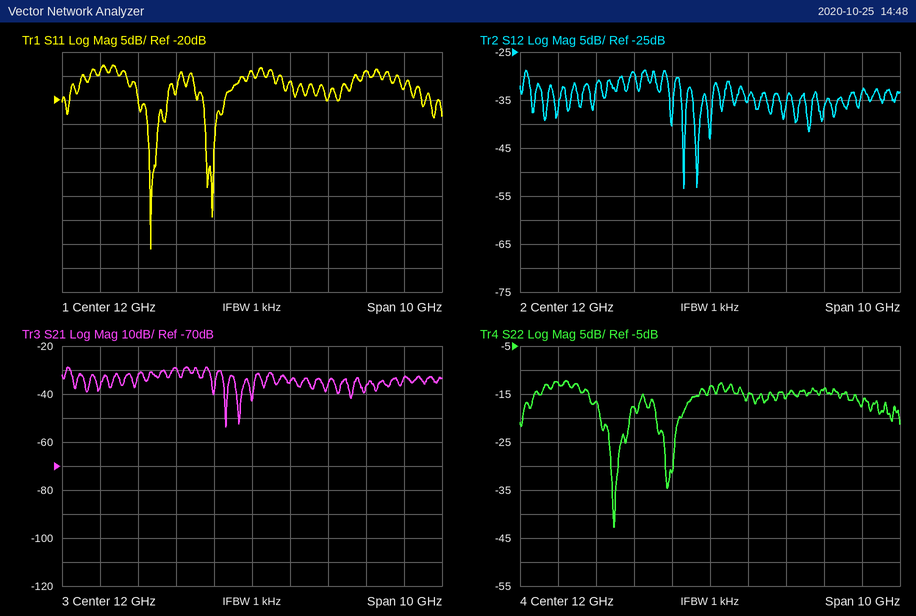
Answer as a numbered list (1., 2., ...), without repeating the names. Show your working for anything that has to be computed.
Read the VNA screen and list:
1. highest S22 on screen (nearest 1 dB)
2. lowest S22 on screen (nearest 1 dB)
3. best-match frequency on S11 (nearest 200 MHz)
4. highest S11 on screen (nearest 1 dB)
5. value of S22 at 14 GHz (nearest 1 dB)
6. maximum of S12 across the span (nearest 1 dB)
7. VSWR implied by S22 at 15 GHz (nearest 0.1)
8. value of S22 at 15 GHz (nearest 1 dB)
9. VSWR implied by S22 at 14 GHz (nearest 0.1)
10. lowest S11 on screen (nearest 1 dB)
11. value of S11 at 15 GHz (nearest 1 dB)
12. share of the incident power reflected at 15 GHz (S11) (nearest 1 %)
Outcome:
1. -12 dB
2. -43 dB
3. 9.4 GHz
4. -13 dB
5. -16 dB
6. -29 dB
7. |Γ| = 10^(-14/20) = 0.1995; VSWR = (1 + 0.1995)/(1 − 0.1995) ≈ 1.5
8. -14 dB
9. |Γ| = 10^(-16/20) = 0.1585; VSWR = (1 + 0.1585)/(1 − 0.1585) ≈ 1.4
10. -51 dB
11. -14 dB
12. 10^(-14/10) ≈ 4 %
